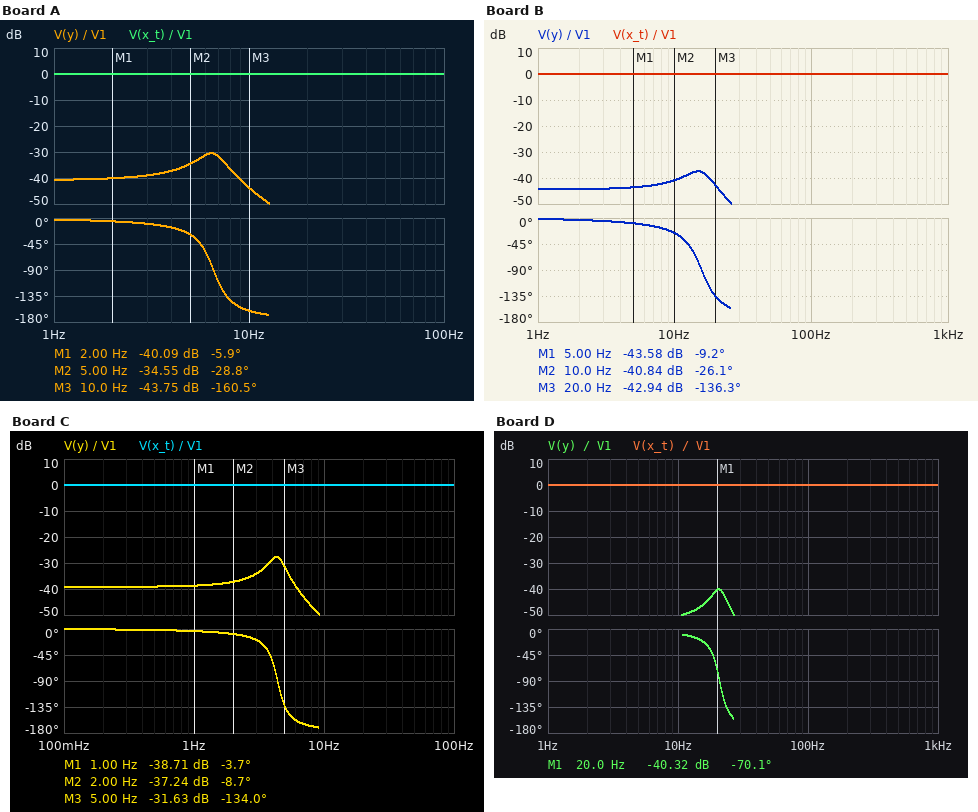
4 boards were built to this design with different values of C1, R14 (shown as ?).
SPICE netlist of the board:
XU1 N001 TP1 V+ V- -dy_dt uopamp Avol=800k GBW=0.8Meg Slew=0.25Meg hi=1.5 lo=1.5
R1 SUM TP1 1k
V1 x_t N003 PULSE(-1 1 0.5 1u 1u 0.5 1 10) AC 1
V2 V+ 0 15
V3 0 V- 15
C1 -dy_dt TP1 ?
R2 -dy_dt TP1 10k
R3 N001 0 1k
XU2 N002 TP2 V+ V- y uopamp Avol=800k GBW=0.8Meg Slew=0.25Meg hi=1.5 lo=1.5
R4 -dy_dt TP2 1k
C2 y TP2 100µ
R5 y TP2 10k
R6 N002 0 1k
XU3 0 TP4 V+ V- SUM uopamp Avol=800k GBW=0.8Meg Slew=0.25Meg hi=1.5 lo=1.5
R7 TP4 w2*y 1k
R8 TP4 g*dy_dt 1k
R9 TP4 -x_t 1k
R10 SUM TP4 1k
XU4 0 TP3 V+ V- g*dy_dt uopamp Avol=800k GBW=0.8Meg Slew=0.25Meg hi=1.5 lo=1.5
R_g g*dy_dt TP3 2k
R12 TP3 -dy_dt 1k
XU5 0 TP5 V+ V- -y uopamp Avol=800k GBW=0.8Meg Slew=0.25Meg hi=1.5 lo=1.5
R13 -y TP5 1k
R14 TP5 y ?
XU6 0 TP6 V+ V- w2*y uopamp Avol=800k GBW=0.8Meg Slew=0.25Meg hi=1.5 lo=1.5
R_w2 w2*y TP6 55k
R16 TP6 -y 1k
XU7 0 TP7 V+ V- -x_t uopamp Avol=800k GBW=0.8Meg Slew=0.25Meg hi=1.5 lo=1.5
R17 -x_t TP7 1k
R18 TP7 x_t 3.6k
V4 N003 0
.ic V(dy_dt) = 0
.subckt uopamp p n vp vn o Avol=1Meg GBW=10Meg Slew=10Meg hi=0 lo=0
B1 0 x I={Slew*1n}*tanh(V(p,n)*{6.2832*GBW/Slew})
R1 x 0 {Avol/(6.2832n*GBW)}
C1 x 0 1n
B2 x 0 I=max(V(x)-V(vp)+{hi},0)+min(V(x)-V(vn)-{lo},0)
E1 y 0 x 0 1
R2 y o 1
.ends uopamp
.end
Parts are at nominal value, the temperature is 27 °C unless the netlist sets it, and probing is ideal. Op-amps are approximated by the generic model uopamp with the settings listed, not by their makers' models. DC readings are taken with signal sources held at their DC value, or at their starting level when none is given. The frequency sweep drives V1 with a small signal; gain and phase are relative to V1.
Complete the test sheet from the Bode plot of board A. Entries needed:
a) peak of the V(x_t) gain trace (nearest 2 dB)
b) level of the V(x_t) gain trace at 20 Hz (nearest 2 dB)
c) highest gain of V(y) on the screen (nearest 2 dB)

0 dB
0 dB
-30 dB
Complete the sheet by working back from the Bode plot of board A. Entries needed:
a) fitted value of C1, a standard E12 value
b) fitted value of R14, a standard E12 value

180 µF
1.8 kΩ
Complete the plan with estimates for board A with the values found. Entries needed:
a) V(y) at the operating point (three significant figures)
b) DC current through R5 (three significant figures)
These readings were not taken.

-9.03 mV
903 nA
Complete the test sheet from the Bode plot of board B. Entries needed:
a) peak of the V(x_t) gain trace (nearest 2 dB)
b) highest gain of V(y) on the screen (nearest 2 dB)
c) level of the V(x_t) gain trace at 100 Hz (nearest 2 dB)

0 dB
-38 dB
0 dB
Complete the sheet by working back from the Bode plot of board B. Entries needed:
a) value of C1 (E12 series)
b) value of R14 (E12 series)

47 µF
1.2 kΩ
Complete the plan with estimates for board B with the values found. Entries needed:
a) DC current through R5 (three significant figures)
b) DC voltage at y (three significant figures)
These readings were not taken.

603 nA
-6.03 mV
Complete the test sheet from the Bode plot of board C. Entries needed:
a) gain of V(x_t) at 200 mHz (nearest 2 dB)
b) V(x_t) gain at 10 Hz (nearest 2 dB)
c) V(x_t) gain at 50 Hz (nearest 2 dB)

0 dB
0 dB
0 dB
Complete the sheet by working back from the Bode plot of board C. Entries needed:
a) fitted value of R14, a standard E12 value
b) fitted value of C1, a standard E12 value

2.2 kΩ
330 µF
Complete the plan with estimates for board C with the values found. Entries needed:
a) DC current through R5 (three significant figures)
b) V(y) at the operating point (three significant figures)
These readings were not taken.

1.10 µA
-11.0 mV
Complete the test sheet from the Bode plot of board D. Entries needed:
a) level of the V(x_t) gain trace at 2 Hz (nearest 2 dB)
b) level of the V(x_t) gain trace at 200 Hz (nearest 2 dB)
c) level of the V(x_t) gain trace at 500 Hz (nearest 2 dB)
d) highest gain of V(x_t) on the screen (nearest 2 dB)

0 dB
0 dB
0 dB
0 dB
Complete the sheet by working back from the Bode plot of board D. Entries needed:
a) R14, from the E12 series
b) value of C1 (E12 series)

470 Ω
68 µF
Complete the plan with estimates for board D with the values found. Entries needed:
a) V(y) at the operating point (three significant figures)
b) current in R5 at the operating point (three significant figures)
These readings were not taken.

-2.37 mV
237 nA
